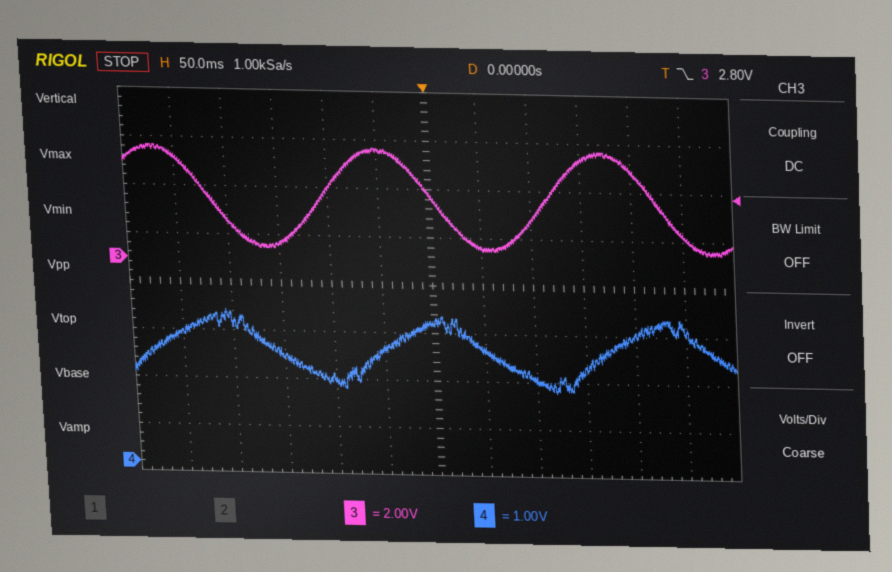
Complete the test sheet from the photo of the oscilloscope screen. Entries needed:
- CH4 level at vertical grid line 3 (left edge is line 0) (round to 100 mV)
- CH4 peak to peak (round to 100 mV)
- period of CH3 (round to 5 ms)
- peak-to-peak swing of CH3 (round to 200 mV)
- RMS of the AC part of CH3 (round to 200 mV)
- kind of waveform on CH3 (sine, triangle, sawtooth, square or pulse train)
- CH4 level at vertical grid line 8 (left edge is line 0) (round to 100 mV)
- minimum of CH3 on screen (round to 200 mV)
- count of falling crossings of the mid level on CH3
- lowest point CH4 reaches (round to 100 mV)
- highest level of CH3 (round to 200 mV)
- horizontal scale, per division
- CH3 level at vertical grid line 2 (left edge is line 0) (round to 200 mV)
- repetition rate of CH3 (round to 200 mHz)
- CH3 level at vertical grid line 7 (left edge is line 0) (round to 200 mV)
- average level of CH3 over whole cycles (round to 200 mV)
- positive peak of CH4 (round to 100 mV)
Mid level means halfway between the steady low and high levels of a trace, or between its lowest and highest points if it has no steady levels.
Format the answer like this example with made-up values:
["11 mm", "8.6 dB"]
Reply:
["2.3 V", "1.6 V", "220 ms", "4.2 V", "1.4 V", "sine", "1.8 V", "400 mV", "3", "1.6 V", "4.6 V", "50 ms", "1.6 V", "4.6 Hz", "600 mV", "2.6 V", "3.2 V"]
